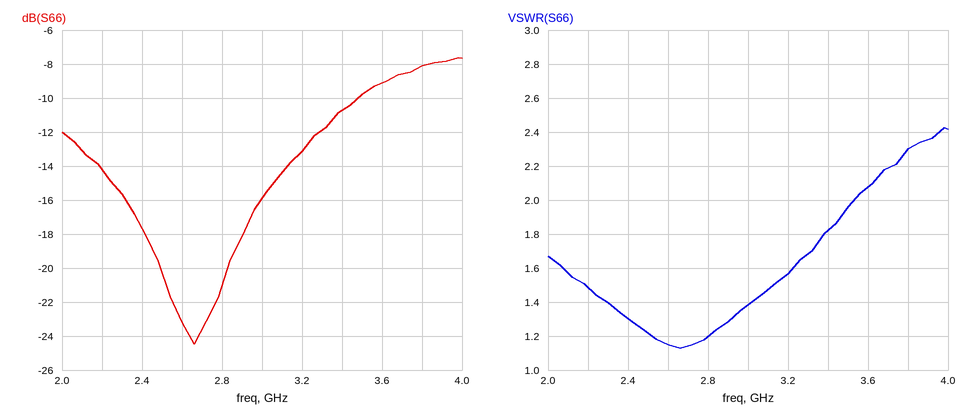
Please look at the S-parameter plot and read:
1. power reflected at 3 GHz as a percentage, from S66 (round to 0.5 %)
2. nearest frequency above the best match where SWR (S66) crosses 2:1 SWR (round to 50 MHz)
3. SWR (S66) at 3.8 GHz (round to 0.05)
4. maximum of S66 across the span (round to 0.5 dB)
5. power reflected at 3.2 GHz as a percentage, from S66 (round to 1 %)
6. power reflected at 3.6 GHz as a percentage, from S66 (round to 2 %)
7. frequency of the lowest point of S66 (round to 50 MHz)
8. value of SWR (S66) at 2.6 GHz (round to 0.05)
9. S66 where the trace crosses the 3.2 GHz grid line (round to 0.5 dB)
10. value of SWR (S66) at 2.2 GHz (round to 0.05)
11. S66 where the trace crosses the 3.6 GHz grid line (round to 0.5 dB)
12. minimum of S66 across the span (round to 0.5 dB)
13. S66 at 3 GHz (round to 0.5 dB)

2.5 %
3.55 GHz
2.30
-7.5 dB
5 %
12 %
2.65 GHz
1.15
-13.0 dB
1.50
-9.0 dB
-24.5 dB
-16.0 dB
